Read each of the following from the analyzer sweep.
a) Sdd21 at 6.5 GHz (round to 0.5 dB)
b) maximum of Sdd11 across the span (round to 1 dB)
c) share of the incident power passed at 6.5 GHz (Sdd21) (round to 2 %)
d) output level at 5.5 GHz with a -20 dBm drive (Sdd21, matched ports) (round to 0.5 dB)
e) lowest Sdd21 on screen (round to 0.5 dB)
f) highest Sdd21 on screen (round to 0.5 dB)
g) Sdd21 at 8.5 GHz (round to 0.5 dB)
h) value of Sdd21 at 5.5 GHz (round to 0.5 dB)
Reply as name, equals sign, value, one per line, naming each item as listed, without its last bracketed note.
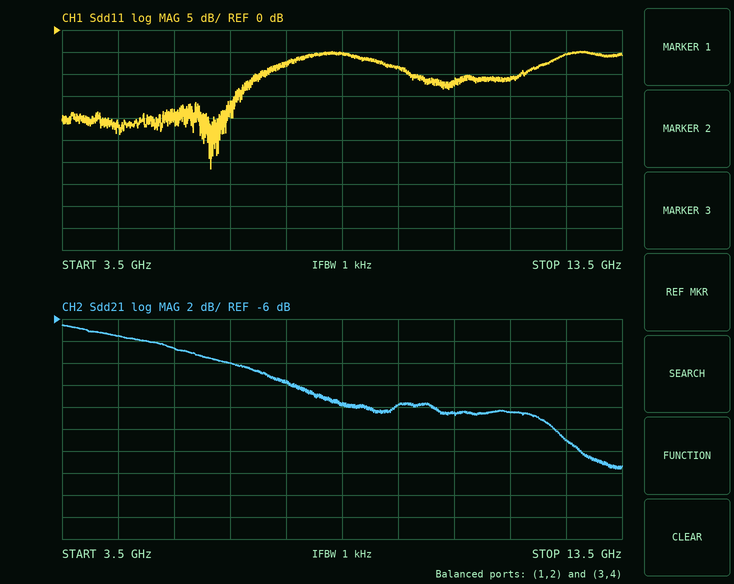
Sdd21 at 6.5 GHz = -10.0 dB
maximum of Sdd11 across the span = -5 dB
share of the incident power passed at 6.5 GHz (Sdd21) = 10 %
output level at 5.5 GHz with a -20 dBm drive (Sdd21, matched ports) = -28.5 dBm
lowest Sdd21 on screen = -19.5 dB
highest Sdd21 on screen = -6.5 dB
Sdd21 at 8.5 GHz = -13.5 dB
value of Sdd21 at 5.5 GHz = -8.5 dB
